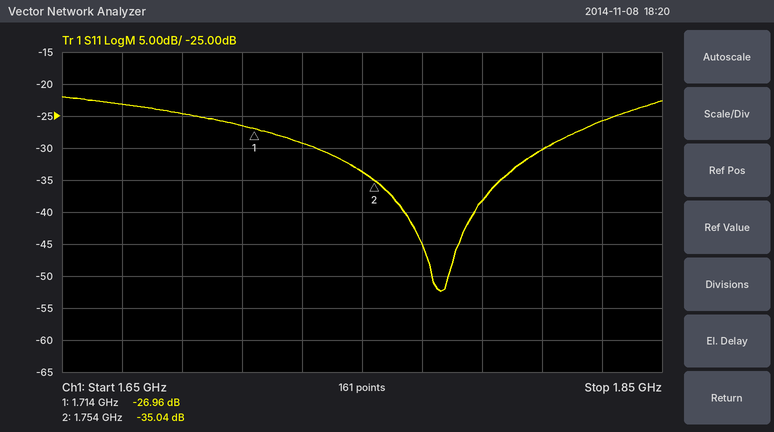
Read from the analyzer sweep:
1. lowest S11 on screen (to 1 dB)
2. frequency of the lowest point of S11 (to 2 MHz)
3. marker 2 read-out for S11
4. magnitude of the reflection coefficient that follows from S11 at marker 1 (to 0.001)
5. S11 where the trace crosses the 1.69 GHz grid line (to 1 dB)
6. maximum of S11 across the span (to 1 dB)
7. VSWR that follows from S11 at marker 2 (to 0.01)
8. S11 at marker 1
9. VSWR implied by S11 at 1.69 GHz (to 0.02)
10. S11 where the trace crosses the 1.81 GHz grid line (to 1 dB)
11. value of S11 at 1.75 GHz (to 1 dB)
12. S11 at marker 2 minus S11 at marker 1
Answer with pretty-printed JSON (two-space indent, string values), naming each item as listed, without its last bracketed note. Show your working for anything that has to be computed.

{
  "lowest S11 on screen": "-52 dB",
  "frequency of the lowest point of S11": "1.776 GHz",
  "marker 2 read-out for S11": "-35.04 dB",
  "magnitude of the reflection coefficient that follows from S11 at marker 1": "10^(-26.96/20) ≈ 0.045",
  "S11 where the trace crosses the 1.69 GHz grid line": "-25 dB",
  "maximum of S11 across the span": "-22 dB",
  "VSWR that follows from S11 at marker 2": "(1 + 0.0177)/(1 − 0.0177) ≈ 1.04",
  "S11 at marker 1": "-26.96 dB",
  "VSWR implied by S11 at 1.69 GHz": "|Γ| = 10^(-25/20) = 0.0562; VSWR = (1 + 0.0562)/(1 − 0.0562) ≈ 1.12",
  "S11 where the trace crosses the 1.81 GHz grid line": "-30 dB",
  "value of S11 at 1.75 GHz": "-34 dB",
  "S11 at marker 2 minus S11 at marker 1": "-35.04 − (-26.96) = -8.08 dB"
}
